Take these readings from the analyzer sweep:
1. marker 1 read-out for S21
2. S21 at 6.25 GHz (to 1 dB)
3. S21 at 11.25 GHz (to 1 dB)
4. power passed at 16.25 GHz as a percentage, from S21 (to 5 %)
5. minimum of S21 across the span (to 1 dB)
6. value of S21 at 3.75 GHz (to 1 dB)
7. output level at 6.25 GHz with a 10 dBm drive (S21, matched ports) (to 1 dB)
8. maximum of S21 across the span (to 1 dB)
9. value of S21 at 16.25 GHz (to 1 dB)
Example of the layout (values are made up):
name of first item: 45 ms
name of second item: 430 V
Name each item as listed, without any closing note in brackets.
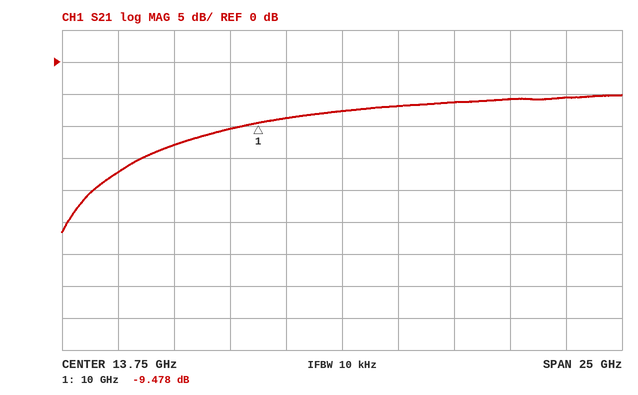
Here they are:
marker 1 read-out for S21: -9.478 dB
S21 at 6.25 GHz: -13 dB
S21 at 11.25 GHz: -9 dB
power passed at 16.25 GHz as a percentage, from S21: 20 %
minimum of S21 across the span: -27 dB
value of S21 at 3.75 GHz: -17 dB
output level at 6.25 GHz with a 10 dBm drive (S21, matched ports): -3 dBm
maximum of S21 across the span: -5 dB
value of S21 at 16.25 GHz: -7 dB
